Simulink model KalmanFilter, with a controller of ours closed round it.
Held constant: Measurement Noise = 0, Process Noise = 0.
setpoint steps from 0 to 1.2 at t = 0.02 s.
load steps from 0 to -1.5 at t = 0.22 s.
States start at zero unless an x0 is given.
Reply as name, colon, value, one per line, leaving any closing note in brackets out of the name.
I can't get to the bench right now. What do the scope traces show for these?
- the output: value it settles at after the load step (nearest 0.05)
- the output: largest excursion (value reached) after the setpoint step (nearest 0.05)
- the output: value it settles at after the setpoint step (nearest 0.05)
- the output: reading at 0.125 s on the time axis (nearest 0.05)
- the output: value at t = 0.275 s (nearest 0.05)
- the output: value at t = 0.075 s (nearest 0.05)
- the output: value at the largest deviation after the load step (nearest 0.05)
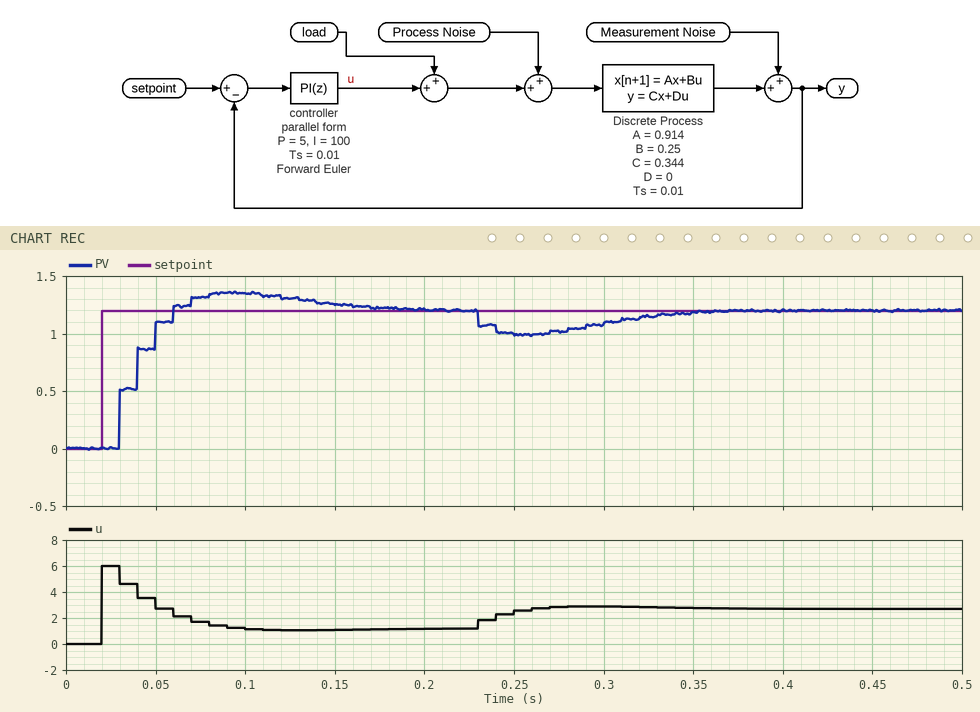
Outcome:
the output: value it settles at after the load step: 1.20
the output: largest excursion (value reached) after the setpoint step: 1.35
the output: value it settles at after the setpoint step: 1.20
the output: reading at 0.125 s on the time axis: 1.30
the output: value at t = 0.275 s: 1.00
the output: value at t = 0.075 s: 1.30
the output: value at the largest deviation after the load step: 1.00
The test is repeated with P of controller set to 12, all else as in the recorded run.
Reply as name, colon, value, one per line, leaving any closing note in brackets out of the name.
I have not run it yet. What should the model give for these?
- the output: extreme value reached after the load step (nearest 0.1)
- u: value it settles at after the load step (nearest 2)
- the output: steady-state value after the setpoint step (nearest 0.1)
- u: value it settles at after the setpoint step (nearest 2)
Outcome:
the output: extreme value reached after the load step: 1.1
u: value it settles at after the load step: 2
the output: steady-state value after the setpoint step: 1.2
u: value it settles at after the setpoint step: 2
